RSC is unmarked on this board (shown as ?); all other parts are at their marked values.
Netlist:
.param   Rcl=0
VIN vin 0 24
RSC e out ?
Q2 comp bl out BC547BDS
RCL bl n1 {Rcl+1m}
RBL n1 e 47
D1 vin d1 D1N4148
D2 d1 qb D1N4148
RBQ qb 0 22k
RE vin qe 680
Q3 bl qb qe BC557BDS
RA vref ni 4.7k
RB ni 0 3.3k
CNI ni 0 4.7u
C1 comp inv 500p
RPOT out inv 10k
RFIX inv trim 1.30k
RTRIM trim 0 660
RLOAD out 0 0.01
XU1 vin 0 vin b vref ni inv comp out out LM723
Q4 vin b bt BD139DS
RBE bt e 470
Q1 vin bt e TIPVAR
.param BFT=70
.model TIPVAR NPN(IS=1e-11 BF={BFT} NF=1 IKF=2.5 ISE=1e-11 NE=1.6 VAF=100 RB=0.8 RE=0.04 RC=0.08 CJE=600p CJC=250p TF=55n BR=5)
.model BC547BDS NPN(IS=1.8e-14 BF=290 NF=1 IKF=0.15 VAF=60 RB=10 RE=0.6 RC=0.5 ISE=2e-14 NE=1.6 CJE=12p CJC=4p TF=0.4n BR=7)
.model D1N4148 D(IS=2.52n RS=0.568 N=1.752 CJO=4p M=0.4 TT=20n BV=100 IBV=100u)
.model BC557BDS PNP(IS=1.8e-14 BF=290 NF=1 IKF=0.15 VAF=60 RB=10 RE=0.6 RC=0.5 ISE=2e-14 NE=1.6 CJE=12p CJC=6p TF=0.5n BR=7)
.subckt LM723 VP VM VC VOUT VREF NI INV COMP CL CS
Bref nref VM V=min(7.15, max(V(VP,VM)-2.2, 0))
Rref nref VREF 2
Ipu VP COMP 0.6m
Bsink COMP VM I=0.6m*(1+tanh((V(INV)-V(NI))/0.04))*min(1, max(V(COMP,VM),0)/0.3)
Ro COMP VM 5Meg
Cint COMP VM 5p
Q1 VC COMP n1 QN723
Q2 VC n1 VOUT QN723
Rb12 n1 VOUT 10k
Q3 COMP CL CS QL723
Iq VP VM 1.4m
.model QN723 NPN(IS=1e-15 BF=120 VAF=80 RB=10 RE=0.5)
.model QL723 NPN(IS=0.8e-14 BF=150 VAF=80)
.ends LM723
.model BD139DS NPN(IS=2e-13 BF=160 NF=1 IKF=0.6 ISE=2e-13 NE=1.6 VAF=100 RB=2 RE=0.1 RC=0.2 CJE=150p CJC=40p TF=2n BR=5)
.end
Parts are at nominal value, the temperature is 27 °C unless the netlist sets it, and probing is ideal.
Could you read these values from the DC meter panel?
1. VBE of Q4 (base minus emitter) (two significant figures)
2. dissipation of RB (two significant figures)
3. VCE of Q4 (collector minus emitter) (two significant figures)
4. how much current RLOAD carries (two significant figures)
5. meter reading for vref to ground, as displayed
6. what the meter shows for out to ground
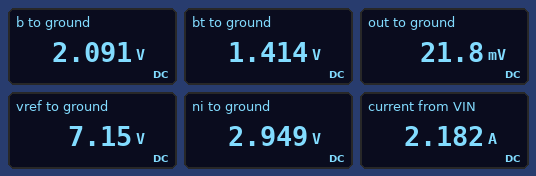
680 mV
2.6 mW
23 V
2.2 A
7.15 V
21.8 mV
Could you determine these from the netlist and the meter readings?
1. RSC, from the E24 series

0.27 Ω
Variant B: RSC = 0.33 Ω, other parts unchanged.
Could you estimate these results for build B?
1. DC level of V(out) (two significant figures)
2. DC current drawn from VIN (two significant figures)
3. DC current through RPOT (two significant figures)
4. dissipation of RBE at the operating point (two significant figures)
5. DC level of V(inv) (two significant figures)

18 mV
1.8 A
1.5 µA
1.3 mW
2.9 mV
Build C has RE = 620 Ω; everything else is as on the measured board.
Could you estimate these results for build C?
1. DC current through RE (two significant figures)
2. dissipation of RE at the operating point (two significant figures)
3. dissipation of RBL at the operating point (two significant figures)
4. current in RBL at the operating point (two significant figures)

880 µA
480 µW
36 µW
870 µA
